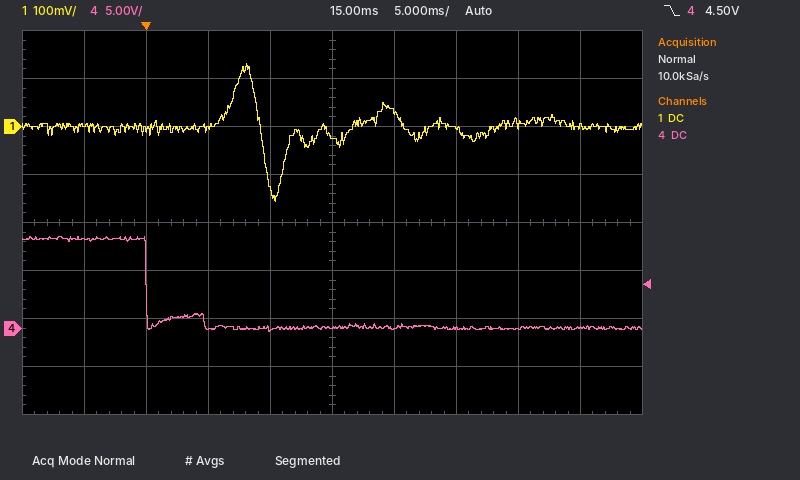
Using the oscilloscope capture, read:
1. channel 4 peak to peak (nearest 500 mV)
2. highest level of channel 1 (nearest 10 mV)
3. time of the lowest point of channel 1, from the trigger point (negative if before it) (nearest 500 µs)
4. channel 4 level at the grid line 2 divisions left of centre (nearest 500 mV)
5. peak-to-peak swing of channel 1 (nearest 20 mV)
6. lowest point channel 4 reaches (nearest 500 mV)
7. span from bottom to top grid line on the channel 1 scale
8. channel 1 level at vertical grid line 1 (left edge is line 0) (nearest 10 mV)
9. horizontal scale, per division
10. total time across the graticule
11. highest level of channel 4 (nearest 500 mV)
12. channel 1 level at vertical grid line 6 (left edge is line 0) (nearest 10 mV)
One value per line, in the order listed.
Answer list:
10.0 V
130 mV
+10.5 ms
0.0 V
280 mV
-500 mV
800 mV
0 mV
5 ms
50 ms
9.5 V
30 mV
